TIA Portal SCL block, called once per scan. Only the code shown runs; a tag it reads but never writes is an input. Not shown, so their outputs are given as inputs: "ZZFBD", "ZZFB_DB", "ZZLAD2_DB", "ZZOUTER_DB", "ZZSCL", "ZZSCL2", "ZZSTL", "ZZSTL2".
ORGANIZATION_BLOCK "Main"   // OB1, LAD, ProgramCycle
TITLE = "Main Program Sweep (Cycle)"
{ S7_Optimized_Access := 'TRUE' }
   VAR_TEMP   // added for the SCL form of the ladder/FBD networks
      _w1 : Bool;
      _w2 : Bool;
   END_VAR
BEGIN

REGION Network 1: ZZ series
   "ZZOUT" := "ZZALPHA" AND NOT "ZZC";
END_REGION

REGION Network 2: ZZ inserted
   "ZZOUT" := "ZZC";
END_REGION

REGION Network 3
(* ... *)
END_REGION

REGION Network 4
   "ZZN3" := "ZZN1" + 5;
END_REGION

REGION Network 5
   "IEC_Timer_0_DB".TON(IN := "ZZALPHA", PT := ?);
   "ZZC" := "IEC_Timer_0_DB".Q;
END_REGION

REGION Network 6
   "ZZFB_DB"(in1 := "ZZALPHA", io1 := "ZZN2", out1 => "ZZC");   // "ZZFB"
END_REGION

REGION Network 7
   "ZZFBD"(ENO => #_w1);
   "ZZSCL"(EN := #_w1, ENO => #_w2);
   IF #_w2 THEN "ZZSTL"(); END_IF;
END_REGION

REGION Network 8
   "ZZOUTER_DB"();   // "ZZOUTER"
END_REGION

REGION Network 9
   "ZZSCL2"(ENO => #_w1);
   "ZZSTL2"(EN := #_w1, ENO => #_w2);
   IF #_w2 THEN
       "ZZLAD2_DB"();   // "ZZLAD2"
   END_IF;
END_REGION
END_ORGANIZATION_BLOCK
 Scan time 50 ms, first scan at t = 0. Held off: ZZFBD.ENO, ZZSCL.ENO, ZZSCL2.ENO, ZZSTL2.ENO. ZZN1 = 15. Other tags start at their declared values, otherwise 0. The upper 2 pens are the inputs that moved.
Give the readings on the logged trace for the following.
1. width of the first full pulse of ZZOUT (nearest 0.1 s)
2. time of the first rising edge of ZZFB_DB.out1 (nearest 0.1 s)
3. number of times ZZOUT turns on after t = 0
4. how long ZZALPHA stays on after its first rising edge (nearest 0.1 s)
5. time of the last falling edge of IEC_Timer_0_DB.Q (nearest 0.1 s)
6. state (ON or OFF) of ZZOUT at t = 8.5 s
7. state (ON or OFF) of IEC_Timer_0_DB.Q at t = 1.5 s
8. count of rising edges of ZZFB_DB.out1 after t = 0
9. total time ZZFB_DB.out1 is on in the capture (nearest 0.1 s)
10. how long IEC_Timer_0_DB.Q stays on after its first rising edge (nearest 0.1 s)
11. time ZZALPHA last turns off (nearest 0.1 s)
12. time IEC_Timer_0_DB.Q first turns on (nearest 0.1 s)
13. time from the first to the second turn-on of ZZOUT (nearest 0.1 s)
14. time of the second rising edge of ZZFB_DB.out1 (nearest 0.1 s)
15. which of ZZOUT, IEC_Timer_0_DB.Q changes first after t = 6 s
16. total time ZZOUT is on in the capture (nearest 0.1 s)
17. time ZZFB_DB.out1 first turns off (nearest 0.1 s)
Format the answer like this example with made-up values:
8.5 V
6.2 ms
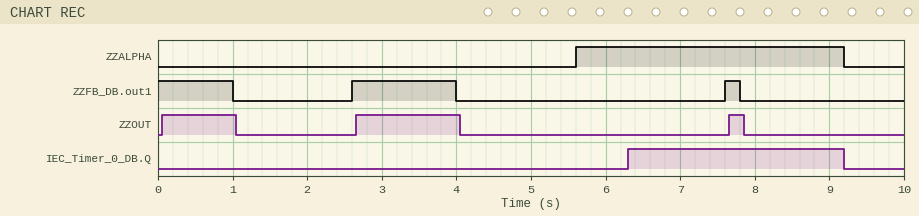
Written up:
1.0 s
2.6 s
3
3.6 s
9.2 s
OFF
OFF
2
2.6 s
2.9 s
9.2 s
6.3 s
2.6 s
7.6 s
IEC_Timer_0_DB.Q
2.6 s
1.0 s
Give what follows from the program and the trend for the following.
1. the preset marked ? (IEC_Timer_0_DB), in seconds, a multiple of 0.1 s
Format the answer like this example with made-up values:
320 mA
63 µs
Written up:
0.7 s
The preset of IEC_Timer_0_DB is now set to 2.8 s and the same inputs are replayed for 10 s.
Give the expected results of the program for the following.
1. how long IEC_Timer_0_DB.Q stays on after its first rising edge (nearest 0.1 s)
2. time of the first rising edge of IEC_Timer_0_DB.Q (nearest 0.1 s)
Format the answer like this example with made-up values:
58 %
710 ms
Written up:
0.8 s
8.4 s
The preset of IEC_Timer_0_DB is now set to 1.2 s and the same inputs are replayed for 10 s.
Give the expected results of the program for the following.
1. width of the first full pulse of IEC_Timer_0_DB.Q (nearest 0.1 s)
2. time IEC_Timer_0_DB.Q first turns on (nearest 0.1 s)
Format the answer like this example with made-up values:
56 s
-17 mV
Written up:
2.4 s
6.8 s
